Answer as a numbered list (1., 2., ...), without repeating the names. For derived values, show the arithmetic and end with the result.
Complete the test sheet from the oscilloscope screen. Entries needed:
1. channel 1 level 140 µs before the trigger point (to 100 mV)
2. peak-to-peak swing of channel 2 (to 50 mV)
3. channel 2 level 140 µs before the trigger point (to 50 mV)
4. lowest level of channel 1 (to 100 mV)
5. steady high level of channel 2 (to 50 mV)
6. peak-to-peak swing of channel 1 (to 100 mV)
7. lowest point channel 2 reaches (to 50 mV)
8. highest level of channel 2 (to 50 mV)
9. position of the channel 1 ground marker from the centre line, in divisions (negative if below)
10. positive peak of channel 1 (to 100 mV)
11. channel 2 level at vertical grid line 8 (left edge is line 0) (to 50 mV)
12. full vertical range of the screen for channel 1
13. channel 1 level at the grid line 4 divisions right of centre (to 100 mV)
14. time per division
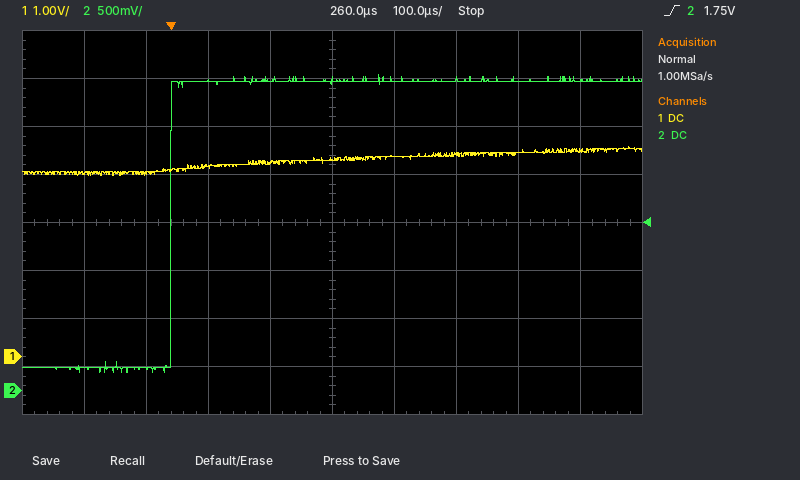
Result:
1. 3.8 V
2. 3.30 V − (200 mV) = 3.10 V
3. 250 mV
4. 3.8 V
5. 3.20 V
6. 4.4 V − (3.8 V) = 600 mV
7. 200 mV
8. 3.30 V
9. -2.8 div
10. 4.4 V
11. 3.20 V
12. 8 V
13. 4.3 V
14. 100 µs
